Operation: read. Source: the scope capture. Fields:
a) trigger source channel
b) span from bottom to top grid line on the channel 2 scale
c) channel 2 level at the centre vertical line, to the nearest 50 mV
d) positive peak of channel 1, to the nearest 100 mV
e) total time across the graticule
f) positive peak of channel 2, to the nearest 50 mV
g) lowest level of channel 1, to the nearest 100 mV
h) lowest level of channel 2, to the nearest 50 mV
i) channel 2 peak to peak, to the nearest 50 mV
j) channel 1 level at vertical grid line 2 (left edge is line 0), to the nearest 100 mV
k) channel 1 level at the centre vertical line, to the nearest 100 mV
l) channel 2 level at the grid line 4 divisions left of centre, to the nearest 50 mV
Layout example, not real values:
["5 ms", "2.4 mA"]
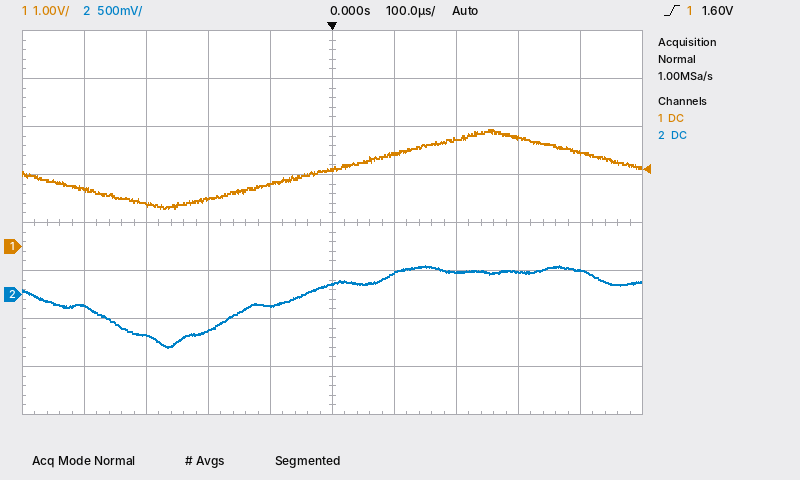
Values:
["channel 1", "4 V", "100 mV", "2.4 V", "1 ms", "300 mV", "800 mV", "-550 mV", "850 mV", "900 mV", "1.6 V", "-100 mV"]
